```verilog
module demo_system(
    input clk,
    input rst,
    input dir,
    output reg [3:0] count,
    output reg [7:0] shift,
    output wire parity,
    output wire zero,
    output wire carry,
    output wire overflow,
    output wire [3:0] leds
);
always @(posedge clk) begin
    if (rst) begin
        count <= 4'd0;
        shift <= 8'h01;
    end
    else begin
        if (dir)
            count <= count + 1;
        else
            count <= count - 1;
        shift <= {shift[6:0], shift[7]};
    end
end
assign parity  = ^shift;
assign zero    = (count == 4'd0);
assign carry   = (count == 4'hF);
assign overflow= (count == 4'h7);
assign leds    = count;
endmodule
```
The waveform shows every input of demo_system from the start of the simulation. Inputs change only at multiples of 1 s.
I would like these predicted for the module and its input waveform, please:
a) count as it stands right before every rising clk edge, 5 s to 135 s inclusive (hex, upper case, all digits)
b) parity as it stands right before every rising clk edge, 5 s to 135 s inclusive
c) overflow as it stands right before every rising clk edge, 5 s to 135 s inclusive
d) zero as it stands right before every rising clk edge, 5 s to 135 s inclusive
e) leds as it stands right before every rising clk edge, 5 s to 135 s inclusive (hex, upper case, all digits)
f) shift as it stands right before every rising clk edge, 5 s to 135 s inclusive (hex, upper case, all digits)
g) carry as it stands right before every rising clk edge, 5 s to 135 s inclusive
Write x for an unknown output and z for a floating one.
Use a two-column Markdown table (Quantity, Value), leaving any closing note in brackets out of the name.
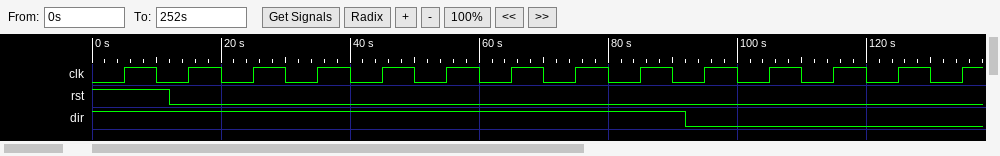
| Quantity | Value |
|---|---|
| count as it stands right before every rising clk edge, 5 s to 135 s inclusive | x, 0, 1, 2, 3, 4, 5, 6, 7, 8, 7, 6, 5, 4 |
| parity as it stands right before every rising clk edge, 5 s to 135 s inclusive | x 1 1 1 1 1 1 1 1 1 1 1 1 1 |
| overflow as it stands right before every rising clk edge, 5 s to 135 s inclusive | x 0 0 0 0 0 0 0 1 0 1 0 0 0 |
| zero as it stands right before every rising clk edge, 5 s to 135 s inclusive | x 1 0 0 0 0 0 0 0 0 0 0 0 0 |
| leds as it stands right before every rising clk edge, 5 s to 135 s inclusive | x, 0, 1, 2, 3, 4, 5, 6, 7, 8, 7, 6, 5, 4 |
| shift as it stands right before every rising clk edge, 5 s to 135 s inclusive | x, 01, 02, 04, 08, 10, 20, 40, 80, 01, 02, 04, 08, 10 |
| carry as it stands right before every rising clk edge, 5 s to 135 s inclusive | x 0 0 0 0 0 0 0 0 0 0 0 0 0 |
